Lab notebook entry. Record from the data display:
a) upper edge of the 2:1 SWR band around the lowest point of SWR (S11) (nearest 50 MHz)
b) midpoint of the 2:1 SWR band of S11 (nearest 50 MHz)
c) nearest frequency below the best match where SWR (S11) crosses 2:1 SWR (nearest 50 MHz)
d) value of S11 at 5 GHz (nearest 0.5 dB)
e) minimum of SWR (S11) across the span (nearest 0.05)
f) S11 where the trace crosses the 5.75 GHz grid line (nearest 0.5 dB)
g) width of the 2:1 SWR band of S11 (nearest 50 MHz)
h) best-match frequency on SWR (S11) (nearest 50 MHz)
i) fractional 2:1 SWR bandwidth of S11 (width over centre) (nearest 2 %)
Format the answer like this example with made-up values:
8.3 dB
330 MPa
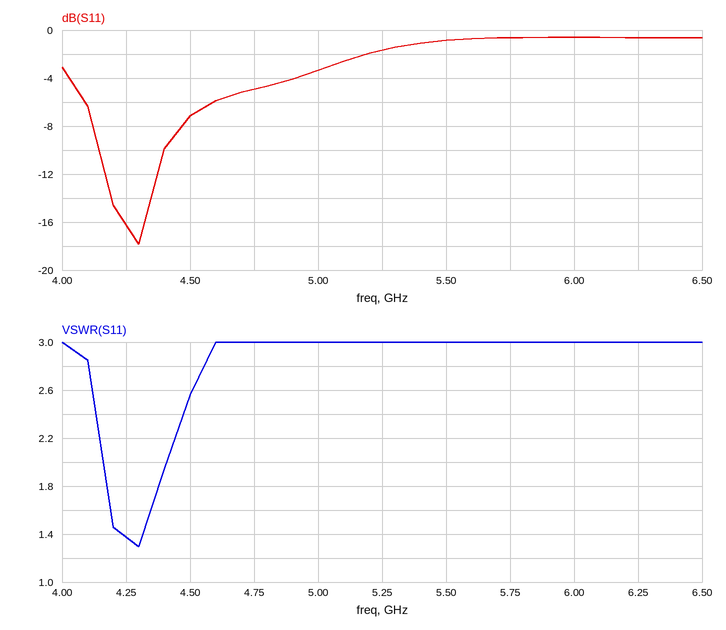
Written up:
4.40 GHz
4.30 GHz
4.15 GHz
-3.5 dB
1.30
-0.5 dB
250 MHz
4.30 GHz
6 %
